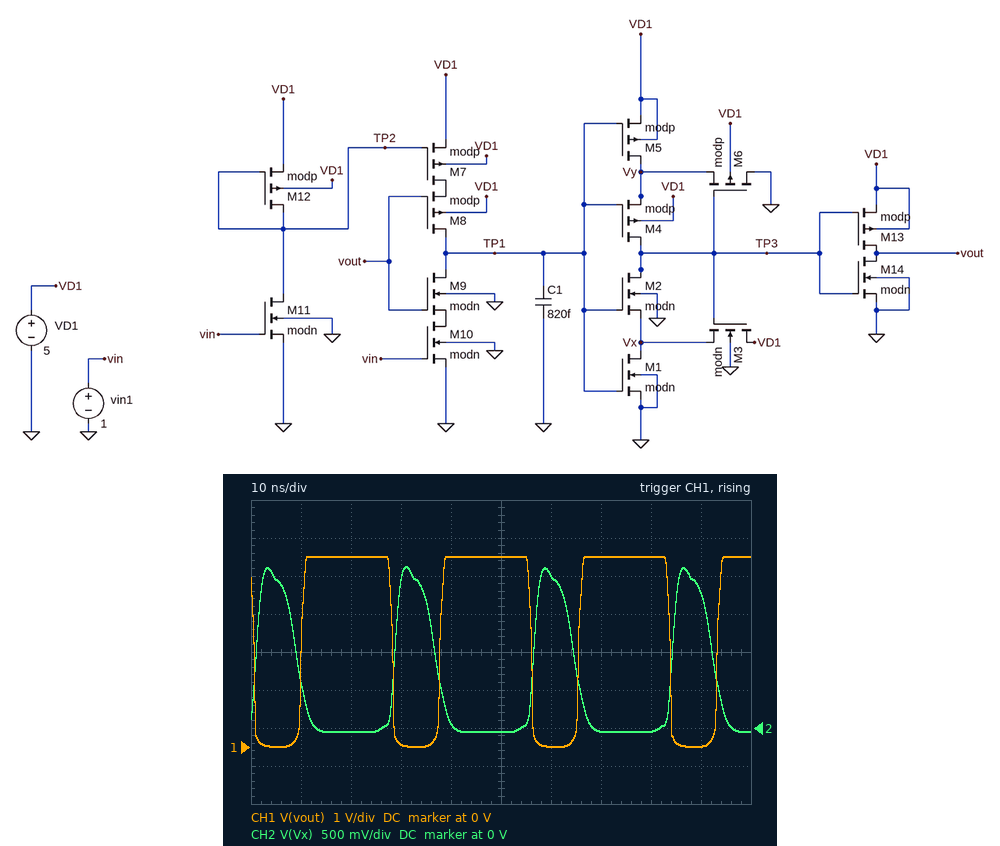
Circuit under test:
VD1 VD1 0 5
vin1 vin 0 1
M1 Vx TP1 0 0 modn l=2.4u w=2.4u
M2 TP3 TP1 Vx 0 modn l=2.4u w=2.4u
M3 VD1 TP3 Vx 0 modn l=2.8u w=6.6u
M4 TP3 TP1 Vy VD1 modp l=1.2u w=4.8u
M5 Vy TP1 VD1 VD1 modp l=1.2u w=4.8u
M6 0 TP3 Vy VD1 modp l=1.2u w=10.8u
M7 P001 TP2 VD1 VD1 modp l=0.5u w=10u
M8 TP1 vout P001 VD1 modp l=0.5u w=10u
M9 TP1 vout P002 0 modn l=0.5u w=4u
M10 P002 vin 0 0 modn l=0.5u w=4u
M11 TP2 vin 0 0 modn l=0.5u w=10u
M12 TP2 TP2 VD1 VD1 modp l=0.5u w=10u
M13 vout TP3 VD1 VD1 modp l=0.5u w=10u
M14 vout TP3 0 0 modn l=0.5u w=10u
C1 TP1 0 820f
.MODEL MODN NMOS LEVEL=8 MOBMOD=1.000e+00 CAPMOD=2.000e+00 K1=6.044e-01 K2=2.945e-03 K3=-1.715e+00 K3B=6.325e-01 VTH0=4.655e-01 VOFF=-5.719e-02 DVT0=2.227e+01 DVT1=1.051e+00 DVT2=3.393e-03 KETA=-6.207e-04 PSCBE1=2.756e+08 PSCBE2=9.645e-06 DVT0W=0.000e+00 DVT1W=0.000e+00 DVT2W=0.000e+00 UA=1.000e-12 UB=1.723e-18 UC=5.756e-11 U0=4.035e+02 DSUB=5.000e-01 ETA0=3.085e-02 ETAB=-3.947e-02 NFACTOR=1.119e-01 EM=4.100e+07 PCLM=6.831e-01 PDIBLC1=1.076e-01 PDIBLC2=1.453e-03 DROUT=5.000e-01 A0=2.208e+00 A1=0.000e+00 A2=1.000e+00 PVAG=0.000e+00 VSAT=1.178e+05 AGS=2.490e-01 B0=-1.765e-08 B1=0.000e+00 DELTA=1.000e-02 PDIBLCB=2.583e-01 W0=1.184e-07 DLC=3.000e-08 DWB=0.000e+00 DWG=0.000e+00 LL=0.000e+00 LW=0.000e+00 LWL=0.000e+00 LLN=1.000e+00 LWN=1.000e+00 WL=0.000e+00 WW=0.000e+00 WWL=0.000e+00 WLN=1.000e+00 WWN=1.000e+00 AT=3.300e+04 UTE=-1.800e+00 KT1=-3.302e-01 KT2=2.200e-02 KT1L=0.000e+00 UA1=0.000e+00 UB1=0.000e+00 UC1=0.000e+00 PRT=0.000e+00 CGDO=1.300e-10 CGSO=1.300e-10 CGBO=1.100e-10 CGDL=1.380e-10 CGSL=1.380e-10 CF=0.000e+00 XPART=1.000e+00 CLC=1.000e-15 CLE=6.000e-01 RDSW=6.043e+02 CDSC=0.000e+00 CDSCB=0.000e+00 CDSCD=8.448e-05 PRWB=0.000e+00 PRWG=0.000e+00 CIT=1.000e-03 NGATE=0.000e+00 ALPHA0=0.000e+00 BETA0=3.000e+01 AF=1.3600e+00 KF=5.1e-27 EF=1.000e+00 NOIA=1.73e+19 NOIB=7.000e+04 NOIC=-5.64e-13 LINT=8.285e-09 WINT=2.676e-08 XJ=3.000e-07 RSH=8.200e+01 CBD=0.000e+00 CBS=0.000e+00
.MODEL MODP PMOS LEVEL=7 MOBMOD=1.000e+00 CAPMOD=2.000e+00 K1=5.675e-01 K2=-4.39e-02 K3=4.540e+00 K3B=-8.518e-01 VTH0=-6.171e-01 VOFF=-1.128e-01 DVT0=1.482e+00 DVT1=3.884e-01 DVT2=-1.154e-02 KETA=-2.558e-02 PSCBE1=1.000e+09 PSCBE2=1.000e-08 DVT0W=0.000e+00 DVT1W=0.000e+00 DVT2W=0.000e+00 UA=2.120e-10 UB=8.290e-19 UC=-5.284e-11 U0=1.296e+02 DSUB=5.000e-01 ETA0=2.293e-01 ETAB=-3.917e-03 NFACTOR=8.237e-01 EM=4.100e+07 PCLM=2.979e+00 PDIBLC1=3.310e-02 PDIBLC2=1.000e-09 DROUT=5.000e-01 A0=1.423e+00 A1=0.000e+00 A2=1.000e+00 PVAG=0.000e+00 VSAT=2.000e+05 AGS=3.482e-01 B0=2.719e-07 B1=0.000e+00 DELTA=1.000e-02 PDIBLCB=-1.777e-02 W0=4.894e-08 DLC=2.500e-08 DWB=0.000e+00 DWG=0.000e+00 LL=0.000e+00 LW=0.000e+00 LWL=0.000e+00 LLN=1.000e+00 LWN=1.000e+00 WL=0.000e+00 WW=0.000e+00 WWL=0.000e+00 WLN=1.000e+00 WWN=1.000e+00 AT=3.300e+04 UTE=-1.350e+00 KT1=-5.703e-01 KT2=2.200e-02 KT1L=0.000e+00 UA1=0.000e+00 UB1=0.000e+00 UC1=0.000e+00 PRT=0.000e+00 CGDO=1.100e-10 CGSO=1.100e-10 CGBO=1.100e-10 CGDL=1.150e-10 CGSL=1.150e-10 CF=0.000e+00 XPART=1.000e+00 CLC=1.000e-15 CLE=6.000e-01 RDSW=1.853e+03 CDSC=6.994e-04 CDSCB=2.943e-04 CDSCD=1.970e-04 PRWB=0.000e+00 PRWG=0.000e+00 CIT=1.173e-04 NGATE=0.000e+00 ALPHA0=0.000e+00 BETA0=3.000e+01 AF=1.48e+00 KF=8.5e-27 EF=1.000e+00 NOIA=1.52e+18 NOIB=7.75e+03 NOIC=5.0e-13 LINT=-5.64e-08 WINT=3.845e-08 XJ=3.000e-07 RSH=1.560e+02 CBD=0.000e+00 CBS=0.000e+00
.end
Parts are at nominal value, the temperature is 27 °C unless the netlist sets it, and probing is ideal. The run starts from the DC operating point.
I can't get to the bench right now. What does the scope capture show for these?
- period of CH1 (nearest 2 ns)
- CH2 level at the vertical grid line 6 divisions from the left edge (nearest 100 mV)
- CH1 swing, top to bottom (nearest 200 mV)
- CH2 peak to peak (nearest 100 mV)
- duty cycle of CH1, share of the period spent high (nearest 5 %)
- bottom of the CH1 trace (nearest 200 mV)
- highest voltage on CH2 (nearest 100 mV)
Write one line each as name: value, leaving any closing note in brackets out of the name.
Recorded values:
period of CH1: 28 ns
CH2 level at the vertical grid line 6 divisions from the left edge: 2.0 V
CH1 swing, top to bottom: 5.0 V
CH2 peak to peak: 2.2 V
duty cycle of CH1, share of the period spent high: 65 %
bottom of the CH1 trace: 0 V
highest voltage on CH2: 2.1 V
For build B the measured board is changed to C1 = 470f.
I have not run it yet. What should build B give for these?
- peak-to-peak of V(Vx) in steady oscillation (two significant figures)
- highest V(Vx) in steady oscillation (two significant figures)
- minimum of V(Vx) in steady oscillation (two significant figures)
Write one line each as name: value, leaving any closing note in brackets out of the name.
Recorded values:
peak-to-peak of V(Vx) in steady oscillation: 1.9 V
highest V(Vx) in steady oscillation: 1.8 V
minimum of V(Vx) in steady oscillation: -90 mV
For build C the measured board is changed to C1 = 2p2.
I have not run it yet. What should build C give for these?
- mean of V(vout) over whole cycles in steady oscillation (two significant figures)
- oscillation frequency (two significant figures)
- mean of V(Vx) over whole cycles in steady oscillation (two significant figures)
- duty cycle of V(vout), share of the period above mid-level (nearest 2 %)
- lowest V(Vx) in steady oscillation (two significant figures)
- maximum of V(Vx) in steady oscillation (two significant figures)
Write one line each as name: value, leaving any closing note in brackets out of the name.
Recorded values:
mean of V(vout) over whole cycles in steady oscillation: 3.4 V
oscillation frequency: 18 MHz
mean of V(Vx) over whole cycles in steady oscillation: 680 mV
duty cycle of V(vout), share of the period above mid-level: 68 %
lowest V(Vx) in steady oscillation: -28 mV
maximum of V(Vx) in steady oscillation: 2.7 V
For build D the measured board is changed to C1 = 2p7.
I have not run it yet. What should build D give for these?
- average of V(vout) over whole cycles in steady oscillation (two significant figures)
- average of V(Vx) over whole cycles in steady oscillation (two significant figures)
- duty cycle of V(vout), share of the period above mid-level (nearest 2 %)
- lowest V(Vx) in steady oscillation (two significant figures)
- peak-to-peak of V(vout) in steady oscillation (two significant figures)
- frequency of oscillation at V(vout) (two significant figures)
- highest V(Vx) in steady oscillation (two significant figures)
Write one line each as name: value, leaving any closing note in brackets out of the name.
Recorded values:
average of V(vout) over whole cycles in steady oscillation: 3.4 V
average of V(Vx) over whole cycles in steady oscillation: 700 mV
duty cycle of V(vout), share of the period above mid-level: 68 %
lowest V(Vx) in steady oscillation: -23 mV
peak-to-peak of V(vout) in steady oscillation: 5.0 V
frequency of oscillation at V(vout): 15 MHz
highest V(Vx) in steady oscillation: 2.8 V
